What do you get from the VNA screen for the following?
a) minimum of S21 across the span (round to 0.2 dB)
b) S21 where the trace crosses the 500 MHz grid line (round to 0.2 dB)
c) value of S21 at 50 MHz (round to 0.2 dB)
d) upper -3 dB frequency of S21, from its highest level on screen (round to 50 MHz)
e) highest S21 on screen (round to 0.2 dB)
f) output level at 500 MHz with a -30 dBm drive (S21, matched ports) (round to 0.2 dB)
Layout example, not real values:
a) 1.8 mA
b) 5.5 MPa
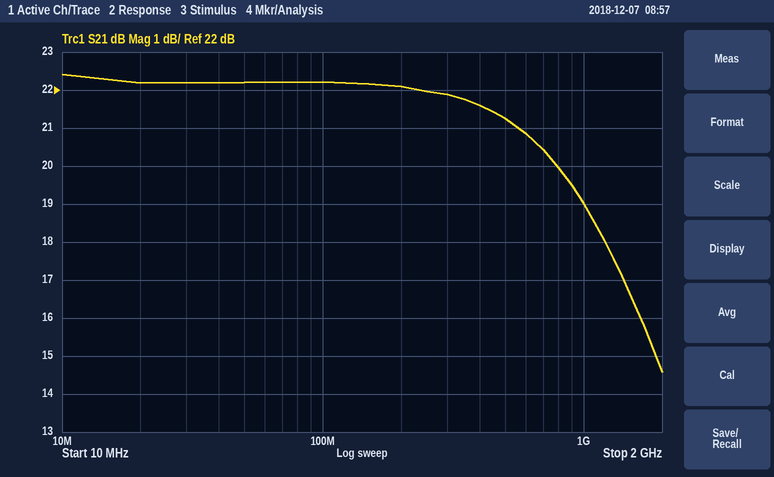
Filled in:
a) 14.6 dB
b) 21.2 dB
c) 22.2 dB
d) 900 MHz
e) 22.4 dB
f) -8.8 dBm
